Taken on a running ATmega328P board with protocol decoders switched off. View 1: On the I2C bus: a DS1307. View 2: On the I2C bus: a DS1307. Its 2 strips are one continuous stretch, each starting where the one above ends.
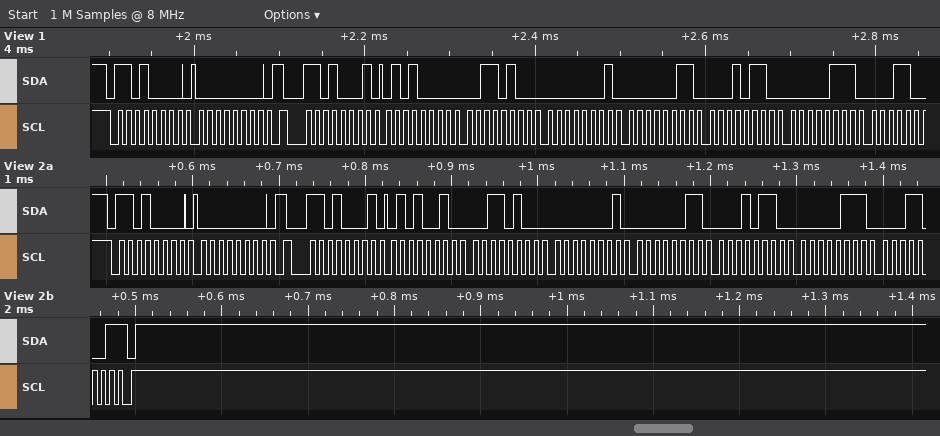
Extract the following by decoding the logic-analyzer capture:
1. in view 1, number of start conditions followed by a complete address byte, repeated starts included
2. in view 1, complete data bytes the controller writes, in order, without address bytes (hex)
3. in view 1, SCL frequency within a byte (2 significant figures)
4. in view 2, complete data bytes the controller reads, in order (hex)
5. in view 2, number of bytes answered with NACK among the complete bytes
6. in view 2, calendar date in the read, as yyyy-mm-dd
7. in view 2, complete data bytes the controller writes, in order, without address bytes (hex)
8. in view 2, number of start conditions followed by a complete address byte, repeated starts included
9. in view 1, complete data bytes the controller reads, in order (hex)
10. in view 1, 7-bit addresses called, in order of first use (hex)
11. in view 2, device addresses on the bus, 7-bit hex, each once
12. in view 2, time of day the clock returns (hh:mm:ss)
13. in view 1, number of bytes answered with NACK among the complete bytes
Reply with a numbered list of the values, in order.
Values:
1. 2
2. 00
3. 100 kHz
4. 52 34 01 03 16 07 19
5. 1
6. 2019-07-16
7. 00
8. 2
9. 50 34 01 03 16 07
10. 0x68
11. 0x68
12. 01:34:52
13. 0
